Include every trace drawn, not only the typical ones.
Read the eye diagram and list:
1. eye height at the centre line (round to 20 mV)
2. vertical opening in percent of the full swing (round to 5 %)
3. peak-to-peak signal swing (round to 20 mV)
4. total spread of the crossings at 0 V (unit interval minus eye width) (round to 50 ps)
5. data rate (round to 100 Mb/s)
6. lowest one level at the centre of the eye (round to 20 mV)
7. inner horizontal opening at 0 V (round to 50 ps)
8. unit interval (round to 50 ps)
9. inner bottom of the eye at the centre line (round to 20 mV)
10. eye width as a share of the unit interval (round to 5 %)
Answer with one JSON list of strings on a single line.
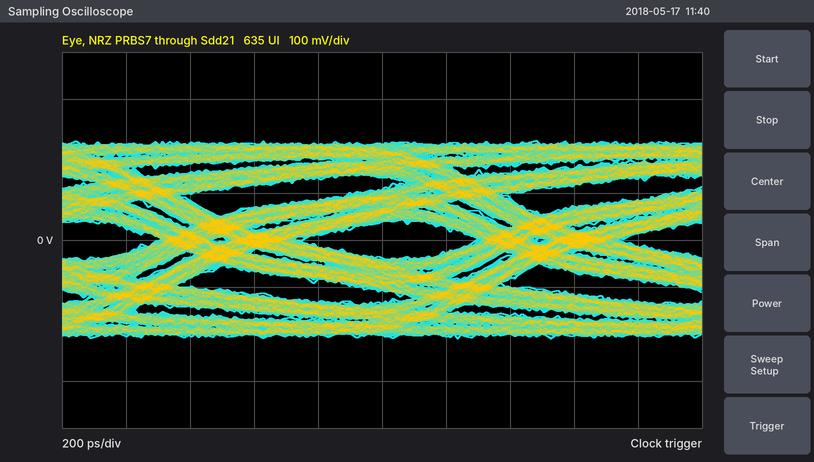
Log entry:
["80 mV", "20 %", "420 mV", "450 ps", "1.0 Gb/s", "40 mV", "550 ps", "1.00 ns", "-40 mV", "55 %"]
